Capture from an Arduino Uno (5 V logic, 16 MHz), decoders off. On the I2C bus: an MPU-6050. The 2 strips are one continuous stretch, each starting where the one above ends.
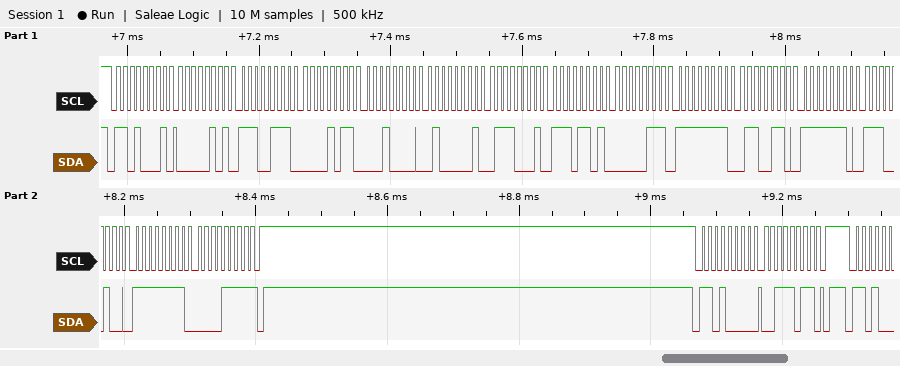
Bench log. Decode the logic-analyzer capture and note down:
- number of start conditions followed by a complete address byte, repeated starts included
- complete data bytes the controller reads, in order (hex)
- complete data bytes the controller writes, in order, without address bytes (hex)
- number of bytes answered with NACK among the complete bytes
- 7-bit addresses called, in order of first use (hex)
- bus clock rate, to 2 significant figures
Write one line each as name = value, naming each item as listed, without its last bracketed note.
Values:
number of start conditions followed by a complete address byte, repeated starts included = 2
complete data bytes the controller reads, in order = 05 E7 0B 10 41 71 ED 07 FF 66 FE E4 FF 0F
complete data bytes the controller writes, in order, without address bytes = 3B
number of bytes answered with NACK among the complete bytes = 1
7-bit addresses called, in order of first use = 0x68
bus clock rate, to 2 significant figures = 100 kHz
